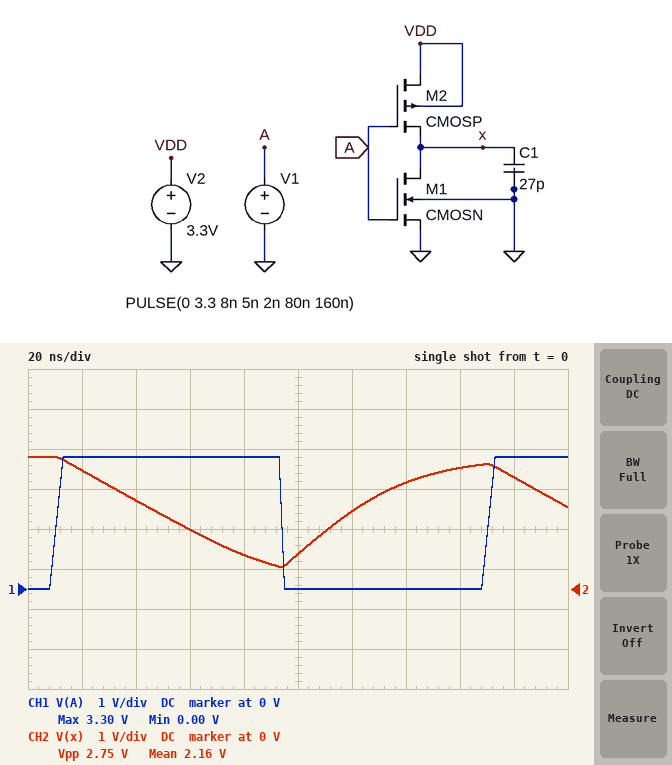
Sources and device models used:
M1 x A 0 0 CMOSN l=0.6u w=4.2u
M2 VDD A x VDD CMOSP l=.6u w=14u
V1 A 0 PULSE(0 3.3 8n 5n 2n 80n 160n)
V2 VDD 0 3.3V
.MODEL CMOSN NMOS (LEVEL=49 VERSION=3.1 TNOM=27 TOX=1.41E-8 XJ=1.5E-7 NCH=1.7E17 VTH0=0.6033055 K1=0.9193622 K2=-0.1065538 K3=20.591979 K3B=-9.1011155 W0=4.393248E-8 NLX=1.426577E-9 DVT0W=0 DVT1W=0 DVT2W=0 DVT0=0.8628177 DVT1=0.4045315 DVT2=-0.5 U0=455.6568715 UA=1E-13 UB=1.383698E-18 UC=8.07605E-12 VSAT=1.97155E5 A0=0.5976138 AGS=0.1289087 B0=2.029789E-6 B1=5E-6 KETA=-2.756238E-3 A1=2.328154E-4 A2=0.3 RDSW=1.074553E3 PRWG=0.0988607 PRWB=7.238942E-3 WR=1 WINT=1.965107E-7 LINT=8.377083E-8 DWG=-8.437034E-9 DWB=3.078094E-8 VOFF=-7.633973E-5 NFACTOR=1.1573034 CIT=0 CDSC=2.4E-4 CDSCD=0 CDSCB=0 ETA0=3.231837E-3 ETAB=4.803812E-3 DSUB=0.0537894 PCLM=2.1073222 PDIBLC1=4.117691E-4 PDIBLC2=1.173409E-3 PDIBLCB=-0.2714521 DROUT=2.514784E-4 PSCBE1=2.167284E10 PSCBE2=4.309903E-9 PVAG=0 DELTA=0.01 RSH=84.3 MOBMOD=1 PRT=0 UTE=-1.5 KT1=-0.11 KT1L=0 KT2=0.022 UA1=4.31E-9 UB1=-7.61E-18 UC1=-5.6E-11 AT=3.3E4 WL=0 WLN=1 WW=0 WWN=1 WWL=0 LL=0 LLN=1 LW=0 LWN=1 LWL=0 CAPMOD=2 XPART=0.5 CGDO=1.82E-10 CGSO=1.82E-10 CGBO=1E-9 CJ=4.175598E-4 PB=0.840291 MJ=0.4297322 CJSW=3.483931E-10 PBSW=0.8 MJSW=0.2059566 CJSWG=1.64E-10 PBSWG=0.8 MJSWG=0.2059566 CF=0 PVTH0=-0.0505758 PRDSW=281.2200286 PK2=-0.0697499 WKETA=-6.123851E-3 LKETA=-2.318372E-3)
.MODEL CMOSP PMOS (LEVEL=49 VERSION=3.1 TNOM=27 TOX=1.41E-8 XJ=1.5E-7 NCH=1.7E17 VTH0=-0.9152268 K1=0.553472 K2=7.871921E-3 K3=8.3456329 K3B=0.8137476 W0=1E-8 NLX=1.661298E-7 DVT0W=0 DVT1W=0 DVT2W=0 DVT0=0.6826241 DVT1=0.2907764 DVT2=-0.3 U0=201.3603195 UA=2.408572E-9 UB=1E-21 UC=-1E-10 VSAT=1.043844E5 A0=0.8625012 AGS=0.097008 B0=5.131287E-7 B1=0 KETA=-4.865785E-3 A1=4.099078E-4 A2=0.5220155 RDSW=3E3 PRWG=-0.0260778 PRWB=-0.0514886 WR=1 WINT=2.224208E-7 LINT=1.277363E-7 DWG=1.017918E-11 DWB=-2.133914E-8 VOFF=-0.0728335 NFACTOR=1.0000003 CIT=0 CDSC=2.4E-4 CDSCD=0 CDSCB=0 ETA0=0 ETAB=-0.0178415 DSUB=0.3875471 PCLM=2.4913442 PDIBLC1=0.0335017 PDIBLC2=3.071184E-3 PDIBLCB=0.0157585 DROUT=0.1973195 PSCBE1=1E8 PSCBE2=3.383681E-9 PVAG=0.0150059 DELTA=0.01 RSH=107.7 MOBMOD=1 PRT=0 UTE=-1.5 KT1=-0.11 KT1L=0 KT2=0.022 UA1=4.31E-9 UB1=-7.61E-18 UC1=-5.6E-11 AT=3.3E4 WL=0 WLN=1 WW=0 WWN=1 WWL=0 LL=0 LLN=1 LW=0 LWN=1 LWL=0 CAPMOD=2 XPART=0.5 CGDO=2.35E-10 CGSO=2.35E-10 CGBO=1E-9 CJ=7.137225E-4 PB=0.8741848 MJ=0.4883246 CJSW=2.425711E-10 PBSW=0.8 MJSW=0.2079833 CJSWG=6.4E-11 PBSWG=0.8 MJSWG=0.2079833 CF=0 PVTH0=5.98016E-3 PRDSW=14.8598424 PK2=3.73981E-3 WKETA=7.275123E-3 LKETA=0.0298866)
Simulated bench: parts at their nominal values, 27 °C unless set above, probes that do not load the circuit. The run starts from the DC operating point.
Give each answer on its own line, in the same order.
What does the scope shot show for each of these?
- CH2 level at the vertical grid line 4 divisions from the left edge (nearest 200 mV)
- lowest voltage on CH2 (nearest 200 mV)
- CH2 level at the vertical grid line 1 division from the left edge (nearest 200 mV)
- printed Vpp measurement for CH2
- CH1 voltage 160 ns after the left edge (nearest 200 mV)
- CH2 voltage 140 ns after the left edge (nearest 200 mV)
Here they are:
800 mV
600 mV
3.0 V
2.75 V
0 V
2.6 V
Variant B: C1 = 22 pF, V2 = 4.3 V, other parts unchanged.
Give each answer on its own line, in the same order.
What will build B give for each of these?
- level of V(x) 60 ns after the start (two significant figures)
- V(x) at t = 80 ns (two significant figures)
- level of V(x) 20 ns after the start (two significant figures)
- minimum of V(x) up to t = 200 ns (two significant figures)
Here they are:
2.0 V
1.2 V
3.9 V
720 mV
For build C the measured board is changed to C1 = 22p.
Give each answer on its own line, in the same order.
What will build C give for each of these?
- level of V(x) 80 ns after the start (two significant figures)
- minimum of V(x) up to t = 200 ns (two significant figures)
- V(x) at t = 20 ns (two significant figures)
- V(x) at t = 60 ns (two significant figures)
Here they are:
510 mV
290 mV
2.9 V
1.1 V
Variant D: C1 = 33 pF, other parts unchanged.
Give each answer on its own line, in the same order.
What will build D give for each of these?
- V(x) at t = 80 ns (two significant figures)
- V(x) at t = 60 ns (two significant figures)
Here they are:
1.2 V
1.8 V
